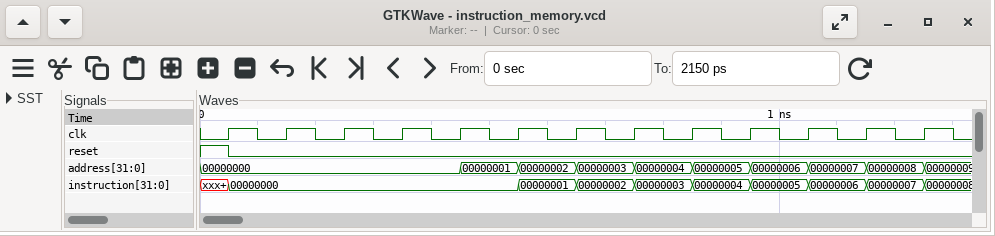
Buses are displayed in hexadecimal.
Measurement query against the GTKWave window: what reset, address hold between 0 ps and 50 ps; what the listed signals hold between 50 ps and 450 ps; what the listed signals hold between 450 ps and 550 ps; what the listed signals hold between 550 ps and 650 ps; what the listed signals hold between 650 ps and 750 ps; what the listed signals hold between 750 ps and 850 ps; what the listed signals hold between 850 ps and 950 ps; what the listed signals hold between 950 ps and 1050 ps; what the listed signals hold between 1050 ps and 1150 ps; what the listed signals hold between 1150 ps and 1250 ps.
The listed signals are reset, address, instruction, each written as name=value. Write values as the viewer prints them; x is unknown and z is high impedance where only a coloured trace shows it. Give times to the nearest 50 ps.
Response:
reset=1, address=00000000
reset=0, address=00000000, instruction=00000000
reset=0, address=00000001, instruction=00000000
reset=0, address=00000002, instruction=00000001
reset=0, address=00000003, instruction=00000002
reset=0, address=00000004, instruction=00000003
reset=0, address=00000005, instruction=00000004
reset=0, address=00000006, instruction=00000005
reset=0, address=00000007, instruction=00000006
reset=0, address=00000008, instruction=00000007
